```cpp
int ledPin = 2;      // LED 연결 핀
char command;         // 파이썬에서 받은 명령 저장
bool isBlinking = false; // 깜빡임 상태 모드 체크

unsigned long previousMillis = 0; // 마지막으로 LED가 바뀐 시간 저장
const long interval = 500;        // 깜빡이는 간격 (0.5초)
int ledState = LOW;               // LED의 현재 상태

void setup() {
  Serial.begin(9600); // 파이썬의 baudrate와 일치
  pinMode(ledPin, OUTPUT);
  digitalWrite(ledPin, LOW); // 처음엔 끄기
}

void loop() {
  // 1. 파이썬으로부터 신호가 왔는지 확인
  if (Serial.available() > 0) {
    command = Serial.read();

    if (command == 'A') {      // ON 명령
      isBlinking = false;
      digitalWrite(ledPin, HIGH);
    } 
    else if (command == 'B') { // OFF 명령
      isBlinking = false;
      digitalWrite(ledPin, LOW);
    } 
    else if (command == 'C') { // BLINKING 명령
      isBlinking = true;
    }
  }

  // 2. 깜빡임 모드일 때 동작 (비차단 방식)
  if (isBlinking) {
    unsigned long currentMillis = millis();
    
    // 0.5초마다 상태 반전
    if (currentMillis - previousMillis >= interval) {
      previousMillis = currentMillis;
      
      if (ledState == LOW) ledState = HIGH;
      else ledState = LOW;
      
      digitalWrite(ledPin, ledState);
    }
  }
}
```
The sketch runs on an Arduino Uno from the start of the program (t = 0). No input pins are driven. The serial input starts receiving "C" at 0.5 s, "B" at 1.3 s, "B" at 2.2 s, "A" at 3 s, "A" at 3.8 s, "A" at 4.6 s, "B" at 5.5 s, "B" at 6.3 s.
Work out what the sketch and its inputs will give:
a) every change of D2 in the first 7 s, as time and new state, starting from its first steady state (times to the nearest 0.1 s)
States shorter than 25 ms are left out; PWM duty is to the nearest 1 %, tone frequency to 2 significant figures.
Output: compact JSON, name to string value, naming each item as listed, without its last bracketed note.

{"every change of D2 in the first 7 s, as time and new state, starting from its first steady state": "0 s low; 0.5 s high; 1 s low; 3 s high; 5.5 s low"}
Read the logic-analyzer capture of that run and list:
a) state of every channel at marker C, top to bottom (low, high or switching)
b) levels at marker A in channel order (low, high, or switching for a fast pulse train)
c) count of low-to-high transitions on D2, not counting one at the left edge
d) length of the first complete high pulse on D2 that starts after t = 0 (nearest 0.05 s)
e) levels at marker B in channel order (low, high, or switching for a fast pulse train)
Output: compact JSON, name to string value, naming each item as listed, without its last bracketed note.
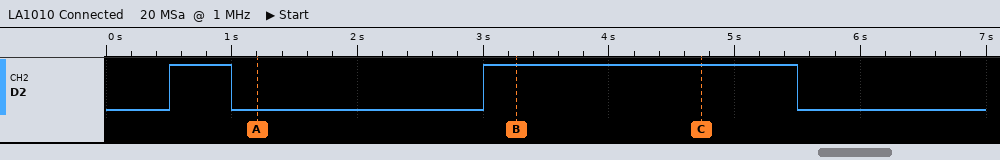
{"state of every channel at marker C, top to bottom": "D2 high", "levels at marker A in channel order": "D2 low", "count of low-to-high transitions on D2, not counting one at the left edge": "2", "length of the first complete high pulse on D2 that starts after t = 0": "0.50 s", "levels at marker B in channel order": "D2 high"}
